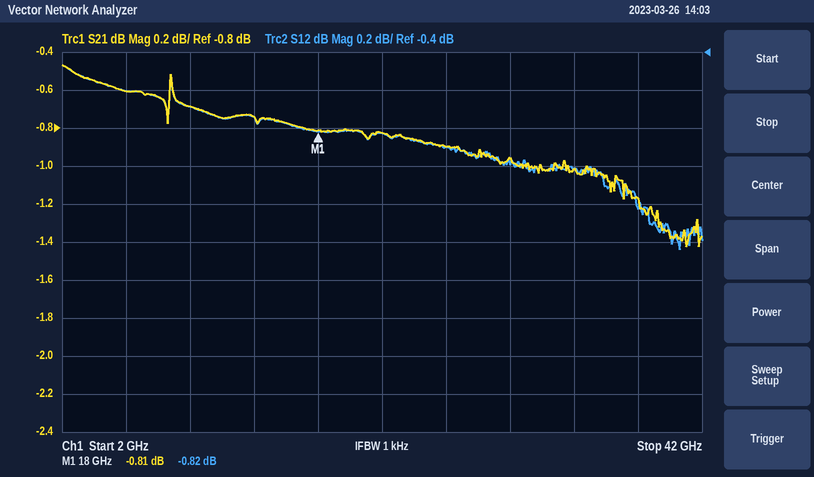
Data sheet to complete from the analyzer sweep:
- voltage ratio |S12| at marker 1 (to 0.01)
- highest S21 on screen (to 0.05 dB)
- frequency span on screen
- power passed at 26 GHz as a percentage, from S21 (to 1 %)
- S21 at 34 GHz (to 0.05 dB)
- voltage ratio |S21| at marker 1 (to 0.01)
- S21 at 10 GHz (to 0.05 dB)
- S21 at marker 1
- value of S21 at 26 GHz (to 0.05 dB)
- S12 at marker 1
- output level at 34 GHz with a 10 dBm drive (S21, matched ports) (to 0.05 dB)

0.91
-0.45 dB
40 GHz
81 %
-1.00 dB
0.91
-0.70 dB
-0.81 dB
-0.90 dB
-0.82 dB
9.00 dBm
